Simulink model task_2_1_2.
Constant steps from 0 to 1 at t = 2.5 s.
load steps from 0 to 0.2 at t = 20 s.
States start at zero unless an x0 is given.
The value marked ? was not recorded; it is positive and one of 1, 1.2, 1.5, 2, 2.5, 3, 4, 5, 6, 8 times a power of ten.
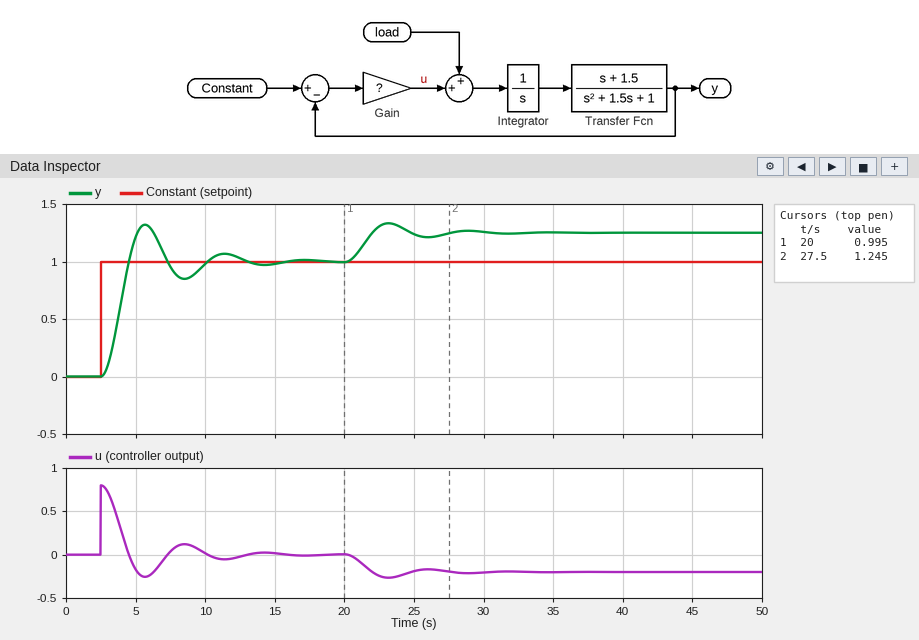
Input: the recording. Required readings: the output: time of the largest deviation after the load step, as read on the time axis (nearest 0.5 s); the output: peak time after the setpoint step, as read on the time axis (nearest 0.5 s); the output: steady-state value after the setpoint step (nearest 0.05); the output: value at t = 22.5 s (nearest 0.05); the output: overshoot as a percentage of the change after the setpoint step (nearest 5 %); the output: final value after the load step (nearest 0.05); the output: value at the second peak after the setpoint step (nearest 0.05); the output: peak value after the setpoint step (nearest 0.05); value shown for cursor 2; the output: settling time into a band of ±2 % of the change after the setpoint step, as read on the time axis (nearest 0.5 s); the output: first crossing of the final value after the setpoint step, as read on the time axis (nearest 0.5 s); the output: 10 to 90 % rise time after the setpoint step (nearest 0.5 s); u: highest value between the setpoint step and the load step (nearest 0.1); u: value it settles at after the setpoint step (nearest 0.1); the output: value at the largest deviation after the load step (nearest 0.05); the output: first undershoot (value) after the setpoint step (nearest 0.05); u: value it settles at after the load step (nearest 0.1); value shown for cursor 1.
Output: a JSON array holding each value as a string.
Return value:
["23.0 s", "5.5 s", "1.00", "1.30", "30 %", "1.25", "1.05", "1.30", "1.245", "15.0 s", "4.5 s", "1.5 s", "0.8", "0.0", "1.35", "0.85", "-0.2", "0.995"]
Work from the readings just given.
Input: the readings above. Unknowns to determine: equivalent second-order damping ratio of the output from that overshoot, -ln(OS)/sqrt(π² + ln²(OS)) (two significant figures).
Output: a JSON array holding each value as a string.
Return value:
["0.36"]
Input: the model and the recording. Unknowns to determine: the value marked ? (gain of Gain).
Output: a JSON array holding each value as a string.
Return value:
["0.8"]
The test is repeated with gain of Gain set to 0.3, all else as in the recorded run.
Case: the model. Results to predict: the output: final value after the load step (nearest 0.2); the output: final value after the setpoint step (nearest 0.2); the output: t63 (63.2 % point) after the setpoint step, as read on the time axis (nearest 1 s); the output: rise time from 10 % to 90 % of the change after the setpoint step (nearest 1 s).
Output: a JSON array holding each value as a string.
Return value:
["1.6", "1.0", "5 s", "3 s"]
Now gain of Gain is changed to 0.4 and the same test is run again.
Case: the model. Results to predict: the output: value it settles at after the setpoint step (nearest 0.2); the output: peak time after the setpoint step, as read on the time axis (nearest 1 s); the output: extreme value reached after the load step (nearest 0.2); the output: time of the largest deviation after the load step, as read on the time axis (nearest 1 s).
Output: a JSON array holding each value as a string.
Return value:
["1.0", "7 s", "1.6", "25 s"]
